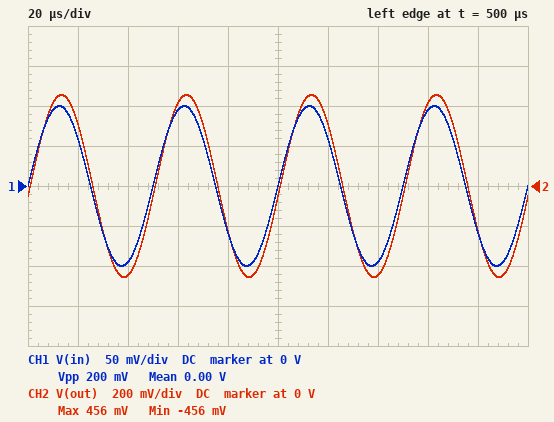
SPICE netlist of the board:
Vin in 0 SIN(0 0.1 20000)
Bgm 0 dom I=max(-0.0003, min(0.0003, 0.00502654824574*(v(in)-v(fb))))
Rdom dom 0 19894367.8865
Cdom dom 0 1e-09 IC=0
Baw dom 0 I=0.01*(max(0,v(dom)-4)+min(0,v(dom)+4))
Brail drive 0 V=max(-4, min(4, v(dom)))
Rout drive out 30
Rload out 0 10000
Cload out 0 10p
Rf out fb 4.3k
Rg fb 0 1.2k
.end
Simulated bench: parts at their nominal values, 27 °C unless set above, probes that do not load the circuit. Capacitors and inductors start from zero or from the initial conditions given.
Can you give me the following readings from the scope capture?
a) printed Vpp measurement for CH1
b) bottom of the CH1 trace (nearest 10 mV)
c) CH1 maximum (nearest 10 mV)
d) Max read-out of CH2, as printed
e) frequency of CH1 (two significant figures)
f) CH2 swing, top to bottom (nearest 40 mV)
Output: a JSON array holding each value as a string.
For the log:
["200 mV", "-100 mV", "100 mV", "456 mV", "20 kHz", "920 mV"]
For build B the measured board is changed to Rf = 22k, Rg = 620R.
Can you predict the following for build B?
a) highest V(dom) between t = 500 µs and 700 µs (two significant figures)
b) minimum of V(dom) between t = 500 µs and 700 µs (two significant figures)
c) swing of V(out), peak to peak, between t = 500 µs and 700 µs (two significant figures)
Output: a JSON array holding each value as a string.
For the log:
["2.6 V", "-2.6 V", "5.3 V"]
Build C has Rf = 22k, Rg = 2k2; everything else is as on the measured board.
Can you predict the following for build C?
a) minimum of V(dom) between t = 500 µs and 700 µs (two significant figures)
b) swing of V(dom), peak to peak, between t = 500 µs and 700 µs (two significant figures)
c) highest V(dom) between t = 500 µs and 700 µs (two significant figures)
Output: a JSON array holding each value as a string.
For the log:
["-1.1 V", "2.1 V", "1.1 V"]
